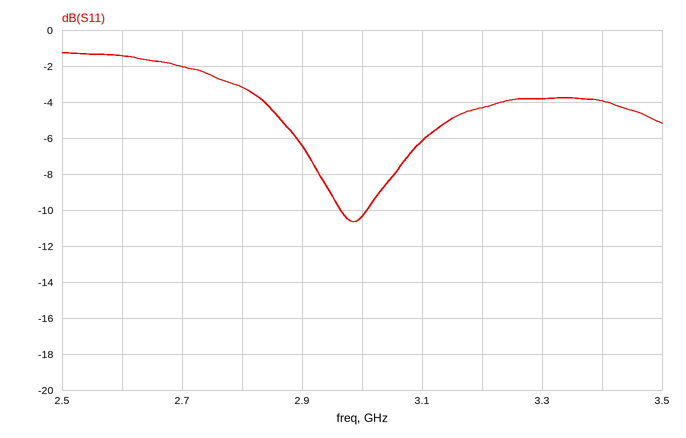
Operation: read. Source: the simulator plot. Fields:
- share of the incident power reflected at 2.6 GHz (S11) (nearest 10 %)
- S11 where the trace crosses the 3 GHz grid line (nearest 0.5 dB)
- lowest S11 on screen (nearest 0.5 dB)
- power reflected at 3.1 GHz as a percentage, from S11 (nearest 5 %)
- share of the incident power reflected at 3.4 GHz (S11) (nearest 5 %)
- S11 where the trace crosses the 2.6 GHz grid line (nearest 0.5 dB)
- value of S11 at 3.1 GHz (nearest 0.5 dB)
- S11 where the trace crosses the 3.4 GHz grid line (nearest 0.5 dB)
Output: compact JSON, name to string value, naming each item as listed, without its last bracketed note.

{"share of the incident power reflected at 2.6 GHz (S11)": "70 %", "S11 where the trace crosses the 3 GHz grid line": "-10.5 dB", "lowest S11 on screen": "-10.5 dB", "power reflected at 3.1 GHz as a percentage, from S11": "25 %", "share of the incident power reflected at 3.4 GHz (S11)": "40 %", "S11 where the trace crosses the 2.6 GHz grid line": "-1.5 dB", "value of S11 at 3.1 GHz": "-6.0 dB", "S11 where the trace crosses the 3.4 GHz grid line": "-4.0 dB"}
